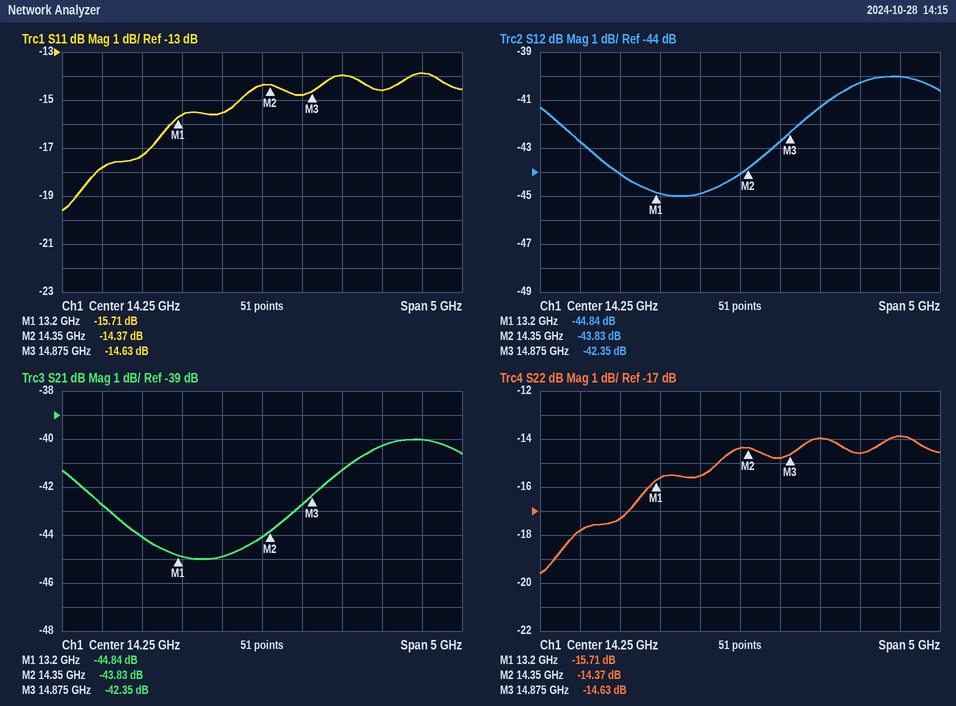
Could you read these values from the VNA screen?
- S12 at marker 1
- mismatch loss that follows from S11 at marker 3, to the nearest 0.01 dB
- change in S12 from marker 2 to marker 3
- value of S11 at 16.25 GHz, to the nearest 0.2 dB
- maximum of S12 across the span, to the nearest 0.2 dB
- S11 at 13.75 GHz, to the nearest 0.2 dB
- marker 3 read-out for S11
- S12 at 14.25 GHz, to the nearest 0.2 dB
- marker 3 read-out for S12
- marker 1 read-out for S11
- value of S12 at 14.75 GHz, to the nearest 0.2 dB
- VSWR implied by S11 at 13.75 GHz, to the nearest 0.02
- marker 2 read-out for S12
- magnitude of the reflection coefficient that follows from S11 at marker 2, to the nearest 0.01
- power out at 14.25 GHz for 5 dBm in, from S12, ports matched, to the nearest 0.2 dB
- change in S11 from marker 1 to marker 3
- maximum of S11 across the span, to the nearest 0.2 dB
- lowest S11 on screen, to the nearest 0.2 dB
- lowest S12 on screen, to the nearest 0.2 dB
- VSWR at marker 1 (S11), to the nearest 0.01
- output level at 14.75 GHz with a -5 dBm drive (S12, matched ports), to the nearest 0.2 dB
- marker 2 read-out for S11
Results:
-44.84 dB
0.15 dB
1.48 dB
-13.8 dB
-40.0 dB
-15.6 dB
-14.63 dB
-44.0 dB
-42.35 dB
-15.71 dB
-42.8 dB
1.40
-43.83 dB
0.19
-39.0 dBm
1.08 dB
-13.8 dB
-19.6 dB
-45.0 dB
1.39
-47.8 dBm
-14.37 dB
